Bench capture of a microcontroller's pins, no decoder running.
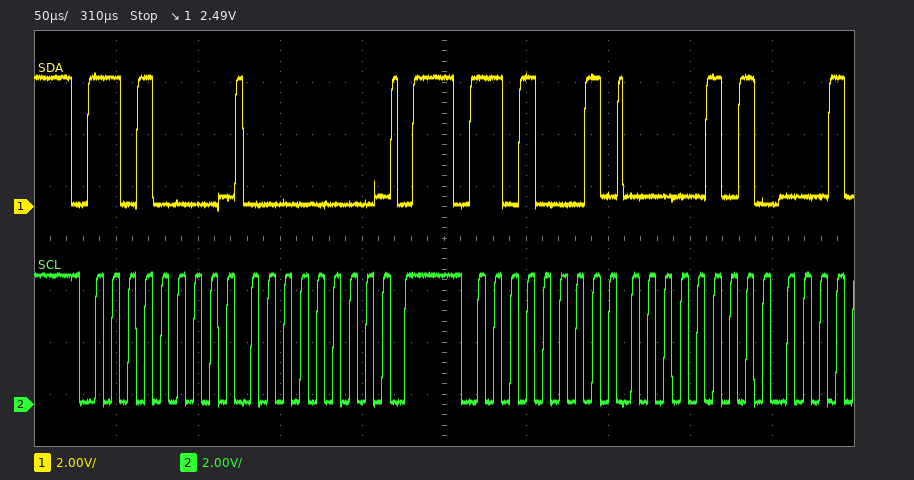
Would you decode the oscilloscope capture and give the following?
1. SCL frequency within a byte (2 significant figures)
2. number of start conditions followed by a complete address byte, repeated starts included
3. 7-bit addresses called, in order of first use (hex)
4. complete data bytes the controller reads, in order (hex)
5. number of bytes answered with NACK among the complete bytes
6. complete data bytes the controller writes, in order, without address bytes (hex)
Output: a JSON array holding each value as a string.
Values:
["100 kHz", "2", "0x68", "05", "0", "00"]
